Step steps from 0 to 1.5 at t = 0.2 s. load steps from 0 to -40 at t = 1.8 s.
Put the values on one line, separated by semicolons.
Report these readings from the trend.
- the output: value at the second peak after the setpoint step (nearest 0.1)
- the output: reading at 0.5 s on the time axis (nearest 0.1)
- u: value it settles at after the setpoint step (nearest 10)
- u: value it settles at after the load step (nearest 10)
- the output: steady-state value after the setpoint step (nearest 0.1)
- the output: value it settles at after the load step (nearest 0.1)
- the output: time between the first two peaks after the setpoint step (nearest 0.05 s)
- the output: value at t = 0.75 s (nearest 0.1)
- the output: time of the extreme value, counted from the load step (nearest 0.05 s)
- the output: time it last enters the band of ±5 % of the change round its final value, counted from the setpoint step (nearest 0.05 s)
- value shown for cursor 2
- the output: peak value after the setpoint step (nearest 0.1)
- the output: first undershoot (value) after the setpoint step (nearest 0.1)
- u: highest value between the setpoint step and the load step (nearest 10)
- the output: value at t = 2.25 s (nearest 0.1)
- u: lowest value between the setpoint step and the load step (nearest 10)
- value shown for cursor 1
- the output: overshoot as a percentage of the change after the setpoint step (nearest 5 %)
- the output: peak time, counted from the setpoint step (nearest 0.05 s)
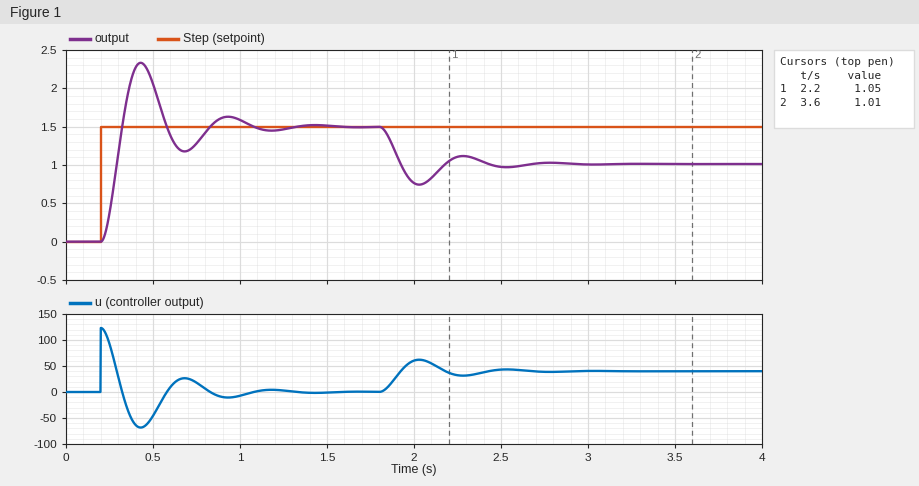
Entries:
1.6; 2.1; 0; 40; 1.5; 1.0; 0.50 s; 1.3; 0.25 s; 0.80 s; 1.01; 2.3; 1.2; 120; 1.1; -70; 1.05; 55 %; 0.25 s
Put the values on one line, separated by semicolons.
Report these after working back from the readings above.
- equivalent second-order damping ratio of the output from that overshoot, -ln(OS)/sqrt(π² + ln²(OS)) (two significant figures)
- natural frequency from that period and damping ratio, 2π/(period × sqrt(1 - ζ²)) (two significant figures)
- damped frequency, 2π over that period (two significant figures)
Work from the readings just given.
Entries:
0.19; 13 rad/s; 13 rad/s
